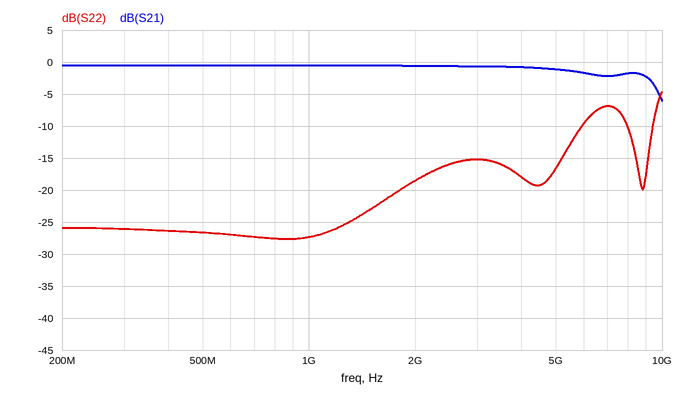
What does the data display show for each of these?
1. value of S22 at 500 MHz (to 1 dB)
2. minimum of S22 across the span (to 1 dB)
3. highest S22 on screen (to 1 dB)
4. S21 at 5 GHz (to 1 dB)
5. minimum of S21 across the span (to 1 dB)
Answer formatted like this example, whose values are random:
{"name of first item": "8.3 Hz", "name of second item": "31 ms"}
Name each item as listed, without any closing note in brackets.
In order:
{"value of S22 at 500 MHz": "-27 dB", "minimum of S22 across the span": "-28 dB", "highest S22 on screen": "-5 dB", "S21 at 5 GHz": "-1 dB", "minimum of S21 across the span": "-6 dB"}
